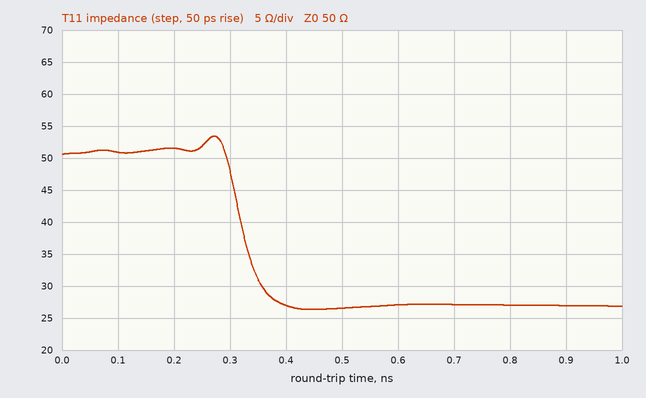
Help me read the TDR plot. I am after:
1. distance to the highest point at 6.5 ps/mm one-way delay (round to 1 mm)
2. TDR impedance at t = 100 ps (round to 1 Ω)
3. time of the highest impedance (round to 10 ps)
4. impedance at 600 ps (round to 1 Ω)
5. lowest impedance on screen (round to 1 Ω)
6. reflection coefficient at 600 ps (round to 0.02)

21 mm
51 Ω
270 ps
27 Ω
26 Ω
-0.30
